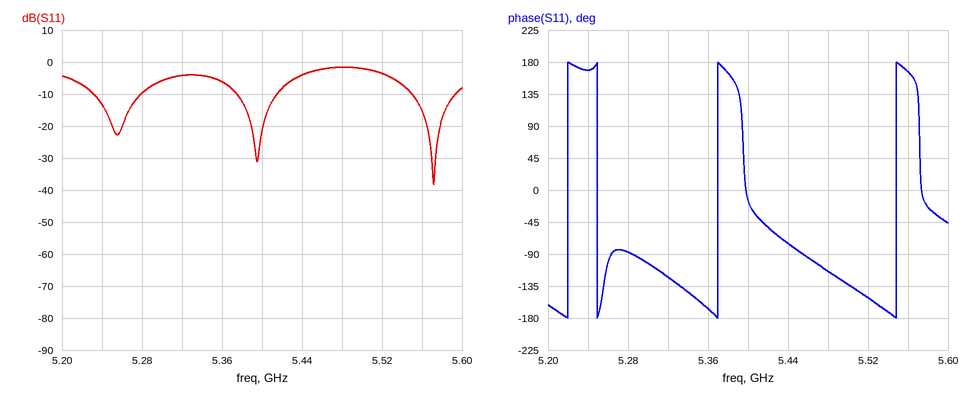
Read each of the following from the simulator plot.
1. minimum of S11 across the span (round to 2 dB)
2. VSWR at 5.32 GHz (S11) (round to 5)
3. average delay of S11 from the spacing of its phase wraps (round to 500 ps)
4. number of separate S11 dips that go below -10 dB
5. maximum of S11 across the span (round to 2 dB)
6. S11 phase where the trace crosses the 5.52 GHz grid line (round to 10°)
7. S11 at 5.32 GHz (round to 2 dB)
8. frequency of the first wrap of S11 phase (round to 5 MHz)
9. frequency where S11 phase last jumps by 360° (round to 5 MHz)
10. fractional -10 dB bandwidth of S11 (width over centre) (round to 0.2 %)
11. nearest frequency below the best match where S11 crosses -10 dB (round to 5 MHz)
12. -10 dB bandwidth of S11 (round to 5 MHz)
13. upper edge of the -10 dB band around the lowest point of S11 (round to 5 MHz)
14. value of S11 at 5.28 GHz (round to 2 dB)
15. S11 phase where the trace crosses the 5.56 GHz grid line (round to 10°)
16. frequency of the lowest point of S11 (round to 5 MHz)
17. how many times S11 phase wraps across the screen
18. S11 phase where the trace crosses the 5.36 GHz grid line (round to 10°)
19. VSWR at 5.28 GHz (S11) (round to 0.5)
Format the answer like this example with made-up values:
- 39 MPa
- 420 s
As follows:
- -38 dB
- 5
- 9.0 ns
- 3
- -2 dB
- -150°
- -4 dB
- 5.220 GHz
- 5.550 GHz
- 0.8 %
- 5.550 GHz
- 45 MHz
- 5.595 GHz
- -10 dB
- 170°
- 5.570 GHz
- 4
- -170°
- 2.0
